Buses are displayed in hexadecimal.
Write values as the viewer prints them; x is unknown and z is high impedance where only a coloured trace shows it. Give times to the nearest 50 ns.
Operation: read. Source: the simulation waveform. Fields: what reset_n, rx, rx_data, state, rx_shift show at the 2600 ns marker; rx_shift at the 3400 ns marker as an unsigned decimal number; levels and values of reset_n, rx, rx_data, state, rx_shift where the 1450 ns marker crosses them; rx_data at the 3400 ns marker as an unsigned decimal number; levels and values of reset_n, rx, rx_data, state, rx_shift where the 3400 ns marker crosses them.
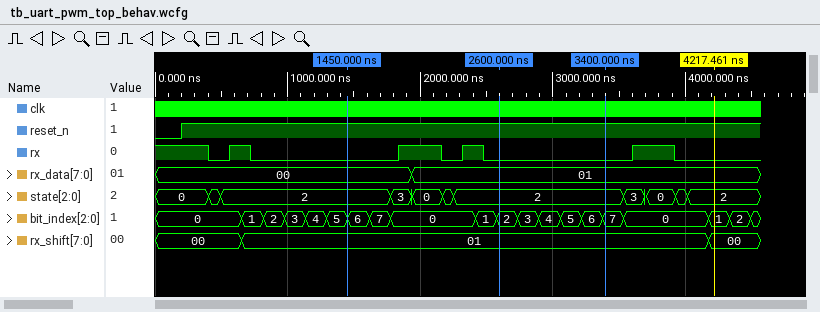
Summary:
reset_n=1, rx=0, rx_data=01, state=2, rx_shift=01
1
reset_n=1, rx=0, rx_data=00, state=2, rx_shift=01
1
reset_n=1, rx=0, rx_data=01, state=2, rx_shift=01
